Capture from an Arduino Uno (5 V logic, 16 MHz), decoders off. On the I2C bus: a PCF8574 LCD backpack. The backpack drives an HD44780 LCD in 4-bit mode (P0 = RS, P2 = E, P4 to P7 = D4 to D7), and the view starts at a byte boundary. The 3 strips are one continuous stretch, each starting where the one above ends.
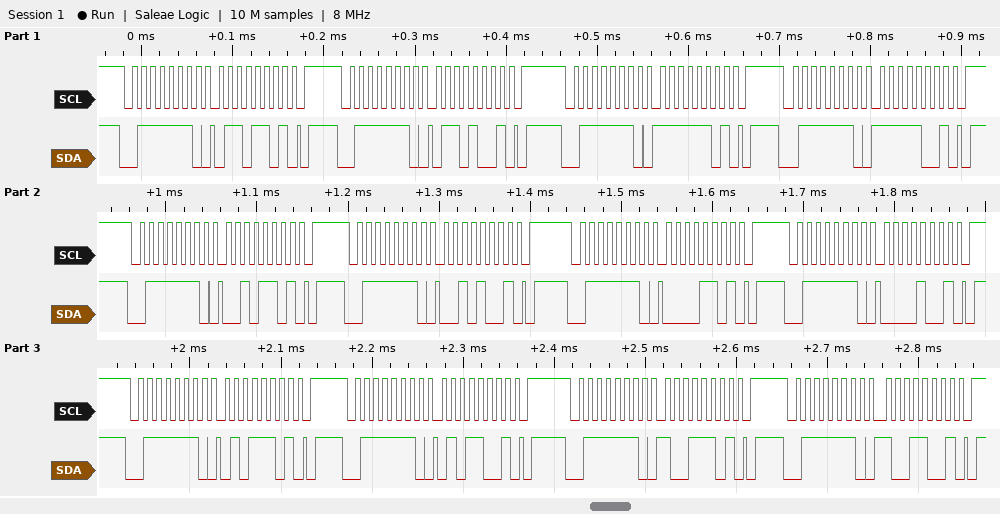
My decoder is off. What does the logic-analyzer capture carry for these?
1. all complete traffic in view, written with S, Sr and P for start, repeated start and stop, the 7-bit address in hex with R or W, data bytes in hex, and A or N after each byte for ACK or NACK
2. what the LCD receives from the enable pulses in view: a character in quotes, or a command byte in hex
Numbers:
S 3FW A 6D A P S 3FW A 69 A P S 3FW A FD A P S 3FW A F9 A P S 3FW A 2D A P S 3FW A 29 A P S 3FW A 0D A P S 3FW A 09 A P S 3FW A 5D A P S 3FW A 59 A P S 3FW A 9D A P S 3FW A 99 A P
'o' ' ' 'Y'
